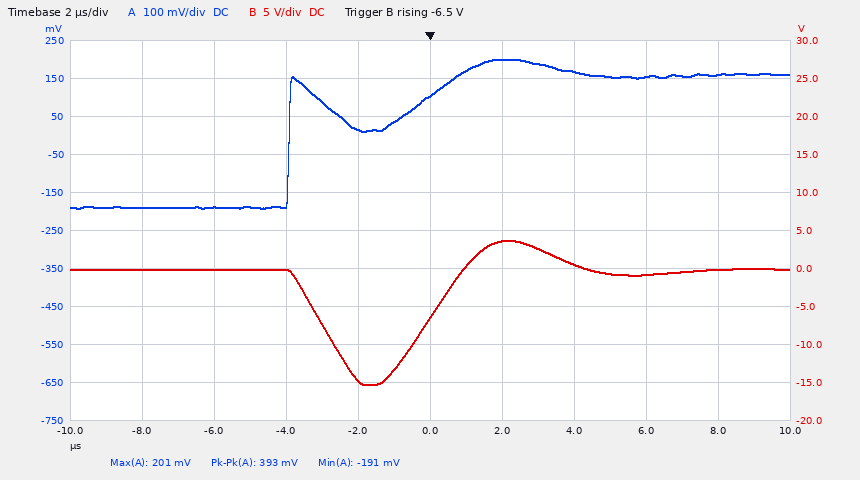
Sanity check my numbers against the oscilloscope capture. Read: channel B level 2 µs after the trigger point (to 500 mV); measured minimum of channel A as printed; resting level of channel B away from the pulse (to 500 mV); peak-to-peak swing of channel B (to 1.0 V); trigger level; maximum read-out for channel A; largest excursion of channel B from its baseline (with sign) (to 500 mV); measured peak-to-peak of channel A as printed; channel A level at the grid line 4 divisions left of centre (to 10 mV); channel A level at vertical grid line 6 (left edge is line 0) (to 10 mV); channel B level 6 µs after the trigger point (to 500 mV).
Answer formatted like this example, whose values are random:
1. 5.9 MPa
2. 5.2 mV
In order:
1. 3.5 V
2. -191 mV
3. 0.0 V
4. 19.0 V
5. -6.5 V
6. 201 mV
7. -15.0 V
8. 393 mV
9. -190 mV
10. 200 mV
11. -1.0 V
